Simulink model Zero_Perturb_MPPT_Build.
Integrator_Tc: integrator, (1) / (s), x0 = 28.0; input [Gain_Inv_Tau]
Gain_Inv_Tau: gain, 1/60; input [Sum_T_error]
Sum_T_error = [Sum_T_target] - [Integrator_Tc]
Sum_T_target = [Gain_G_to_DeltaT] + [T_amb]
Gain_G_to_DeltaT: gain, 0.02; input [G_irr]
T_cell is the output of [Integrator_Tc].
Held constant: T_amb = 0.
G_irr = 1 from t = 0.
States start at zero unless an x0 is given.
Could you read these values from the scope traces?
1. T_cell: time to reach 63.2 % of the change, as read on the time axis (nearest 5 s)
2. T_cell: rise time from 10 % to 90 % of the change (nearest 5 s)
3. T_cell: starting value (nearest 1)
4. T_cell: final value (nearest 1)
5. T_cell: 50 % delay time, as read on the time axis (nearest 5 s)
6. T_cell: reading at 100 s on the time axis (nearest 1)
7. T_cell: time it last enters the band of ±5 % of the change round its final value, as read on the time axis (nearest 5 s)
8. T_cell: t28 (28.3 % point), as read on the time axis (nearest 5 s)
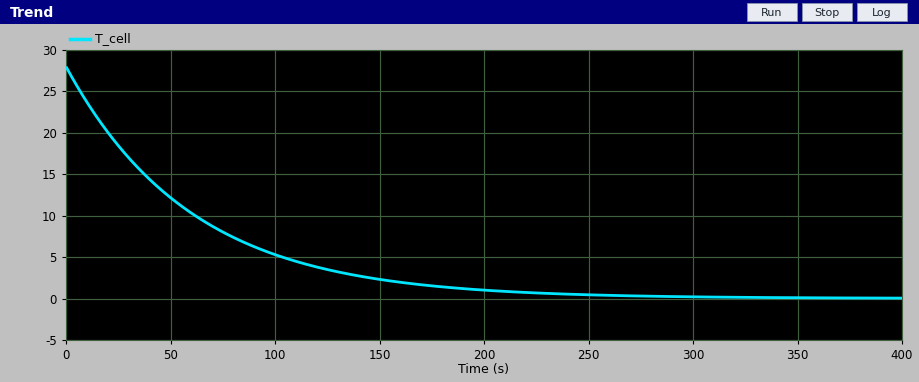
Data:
60 s
130 s
28
0
40 s
5
180 s
20 s
